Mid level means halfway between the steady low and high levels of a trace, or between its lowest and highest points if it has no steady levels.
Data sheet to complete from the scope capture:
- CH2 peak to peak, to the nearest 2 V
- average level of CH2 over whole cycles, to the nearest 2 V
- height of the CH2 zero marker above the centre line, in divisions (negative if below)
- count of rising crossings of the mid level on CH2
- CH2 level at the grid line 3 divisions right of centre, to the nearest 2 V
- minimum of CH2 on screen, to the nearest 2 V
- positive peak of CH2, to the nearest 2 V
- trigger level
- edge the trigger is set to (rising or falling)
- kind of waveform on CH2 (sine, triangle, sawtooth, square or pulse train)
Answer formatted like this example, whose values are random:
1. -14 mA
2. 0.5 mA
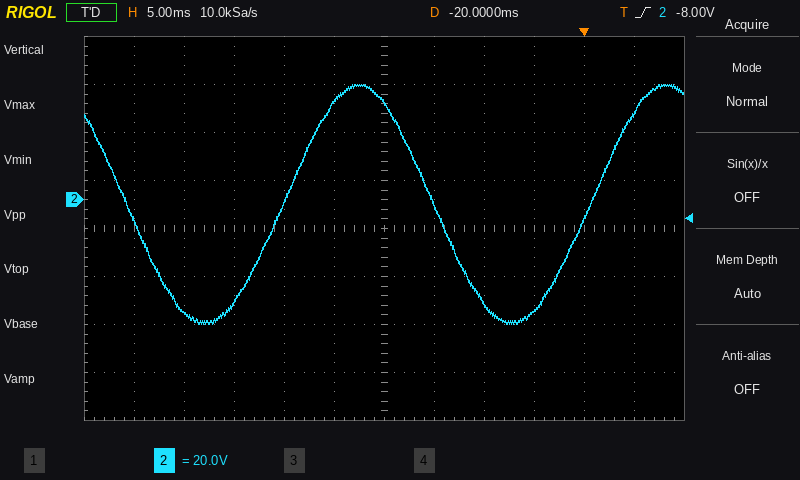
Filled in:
1. 100 V
2. -2 V
3. +0.6 div
4. 2
5. -46 V
6. -52 V
7. 48 V
8. -8.00 V
9. rising
10. sine
